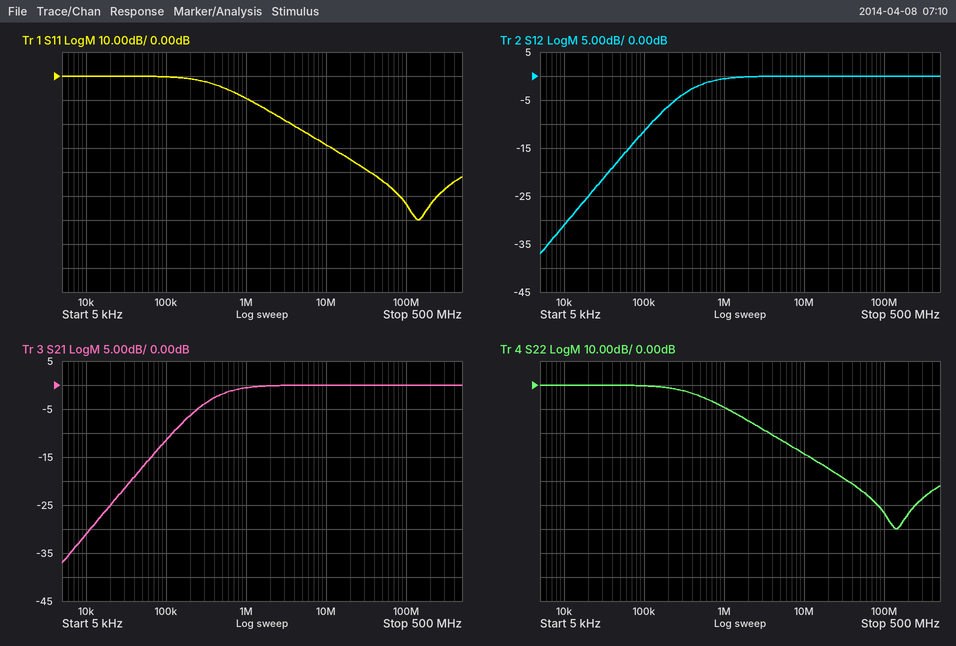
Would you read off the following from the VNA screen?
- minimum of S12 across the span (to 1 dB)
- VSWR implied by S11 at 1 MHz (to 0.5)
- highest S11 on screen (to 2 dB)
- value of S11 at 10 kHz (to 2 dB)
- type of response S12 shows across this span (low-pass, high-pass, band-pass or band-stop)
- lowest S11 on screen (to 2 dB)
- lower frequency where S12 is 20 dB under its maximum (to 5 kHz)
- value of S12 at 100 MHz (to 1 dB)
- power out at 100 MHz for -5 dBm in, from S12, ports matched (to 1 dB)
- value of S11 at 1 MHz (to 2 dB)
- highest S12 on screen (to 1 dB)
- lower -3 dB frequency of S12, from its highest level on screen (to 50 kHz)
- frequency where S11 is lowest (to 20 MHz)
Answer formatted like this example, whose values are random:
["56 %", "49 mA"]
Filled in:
["-37 dB", "2.0", "0 dB", "0 dB", "high-pass", "-60 dB", "35 kHz", "0 dB", "-5 dBm", "-10 dB", "0 dB", "350 kHz", "140 MHz"]
